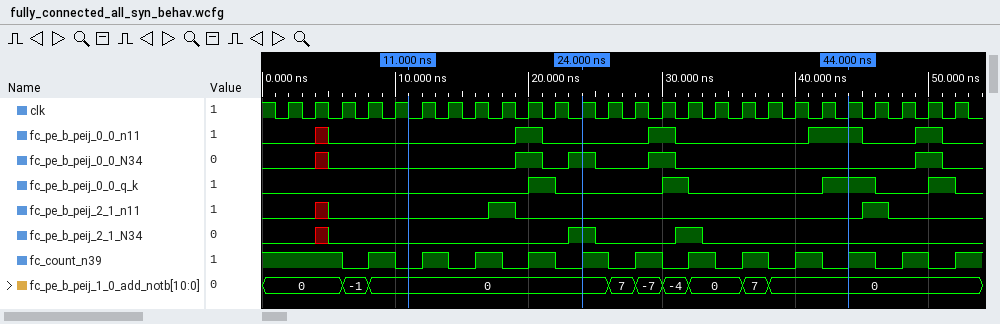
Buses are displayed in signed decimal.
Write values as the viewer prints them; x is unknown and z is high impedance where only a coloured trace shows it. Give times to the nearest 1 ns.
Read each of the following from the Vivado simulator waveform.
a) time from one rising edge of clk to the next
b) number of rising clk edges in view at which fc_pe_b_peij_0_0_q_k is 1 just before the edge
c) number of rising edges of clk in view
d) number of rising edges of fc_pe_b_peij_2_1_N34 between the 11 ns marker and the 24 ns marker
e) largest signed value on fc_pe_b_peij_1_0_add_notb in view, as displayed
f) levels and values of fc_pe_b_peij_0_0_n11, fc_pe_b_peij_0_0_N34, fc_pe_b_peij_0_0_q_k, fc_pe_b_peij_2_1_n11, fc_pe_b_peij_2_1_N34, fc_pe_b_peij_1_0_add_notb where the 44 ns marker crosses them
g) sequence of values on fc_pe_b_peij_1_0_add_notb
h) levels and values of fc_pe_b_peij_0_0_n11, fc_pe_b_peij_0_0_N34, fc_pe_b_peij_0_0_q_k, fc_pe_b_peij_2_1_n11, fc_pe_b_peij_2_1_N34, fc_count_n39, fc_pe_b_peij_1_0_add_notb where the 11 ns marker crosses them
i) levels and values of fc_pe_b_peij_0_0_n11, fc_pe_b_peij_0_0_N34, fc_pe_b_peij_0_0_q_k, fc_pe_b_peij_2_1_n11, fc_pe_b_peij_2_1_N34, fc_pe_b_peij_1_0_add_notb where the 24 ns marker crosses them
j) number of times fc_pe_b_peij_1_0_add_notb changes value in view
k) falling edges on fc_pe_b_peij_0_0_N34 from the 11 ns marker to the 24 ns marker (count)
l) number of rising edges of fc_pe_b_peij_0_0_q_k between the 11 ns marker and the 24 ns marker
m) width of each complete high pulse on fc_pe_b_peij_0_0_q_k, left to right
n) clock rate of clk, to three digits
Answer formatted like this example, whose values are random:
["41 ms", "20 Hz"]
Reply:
["2 ns", "5", "26", "1", "7", "fc_pe_b_peij_0_0_n11=1, fc_pe_b_peij_0_0_N34=0, fc_pe_b_peij_0_0_q_k=1, fc_pe_b_peij_2_1_n11=0, fc_pe_b_peij_2_1_N34=0, fc_pe_b_peij_1_0_add_notb=0", "0, -1, 0, 7, -7, -4, 0, 7, 0", "fc_pe_b_peij_0_0_n11=0, fc_pe_b_peij_0_0_N34=0, fc_pe_b_peij_0_0_q_k=0, fc_pe_b_peij_2_1_n11=0, fc_pe_b_peij_2_1_N34=0, fc_count_n39=0, fc_pe_b_peij_1_0_add_notb=0", "fc_pe_b_peij_0_0_n11=0, fc_pe_b_peij_0_0_N34=1, fc_pe_b_peij_0_0_q_k=0, fc_pe_b_peij_2_1_n11=0, fc_pe_b_peij_2_1_N34=1, fc_pe_b_peij_1_0_add_notb=0", "8", "1", "1", "2 ns, 2 ns, 4 ns, 2 ns", "500 MHz"]
